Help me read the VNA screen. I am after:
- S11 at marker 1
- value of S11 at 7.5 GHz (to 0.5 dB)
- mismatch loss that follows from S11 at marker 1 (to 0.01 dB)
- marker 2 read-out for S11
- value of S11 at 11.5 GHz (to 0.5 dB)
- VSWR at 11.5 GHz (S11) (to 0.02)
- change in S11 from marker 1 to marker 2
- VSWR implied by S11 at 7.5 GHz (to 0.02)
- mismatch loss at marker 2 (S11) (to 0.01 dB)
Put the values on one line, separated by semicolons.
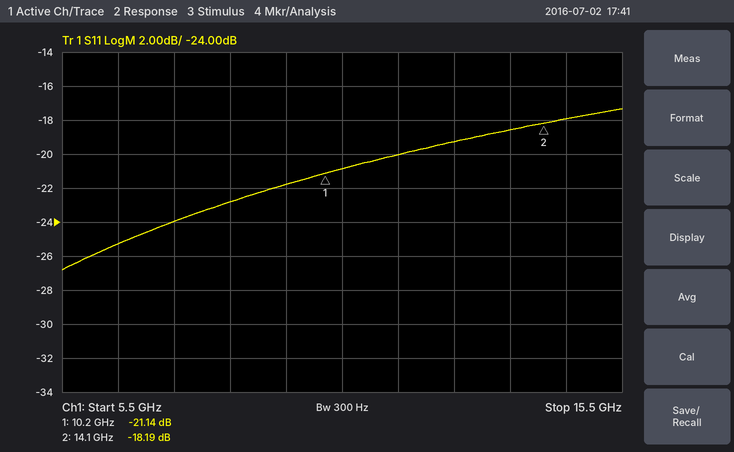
-21.14 dB; -24.0 dB; 0.03 dB; -18.19 dB; -20.0 dB; 1.22; 2.95 dB; 1.14; 0.07 dB
